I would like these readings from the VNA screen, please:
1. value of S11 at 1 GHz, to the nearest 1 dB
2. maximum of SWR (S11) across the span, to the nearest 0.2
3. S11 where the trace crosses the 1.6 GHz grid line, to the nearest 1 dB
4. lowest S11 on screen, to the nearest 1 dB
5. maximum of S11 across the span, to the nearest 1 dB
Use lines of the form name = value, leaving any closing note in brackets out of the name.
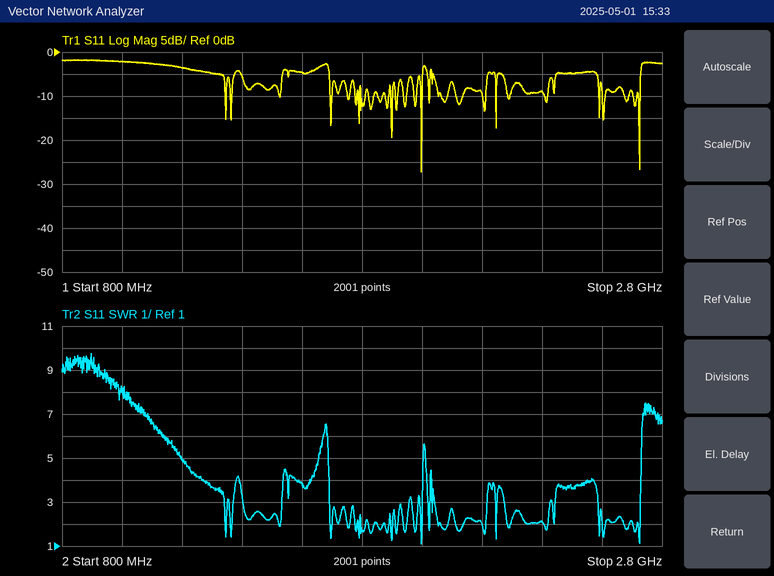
value of S11 at 1 GHz, to the nearest 1 dB = -2 dB
maximum of SWR (S11) across the span, to the nearest 0.2 = 9.8
S11 where the trace crosses the 1.6 GHz grid line, to the nearest 1 dB = -5 dB
lowest S11 on screen, to the nearest 1 dB = -27 dB
maximum of S11 across the span, to the nearest 1 dB = -2 dB
